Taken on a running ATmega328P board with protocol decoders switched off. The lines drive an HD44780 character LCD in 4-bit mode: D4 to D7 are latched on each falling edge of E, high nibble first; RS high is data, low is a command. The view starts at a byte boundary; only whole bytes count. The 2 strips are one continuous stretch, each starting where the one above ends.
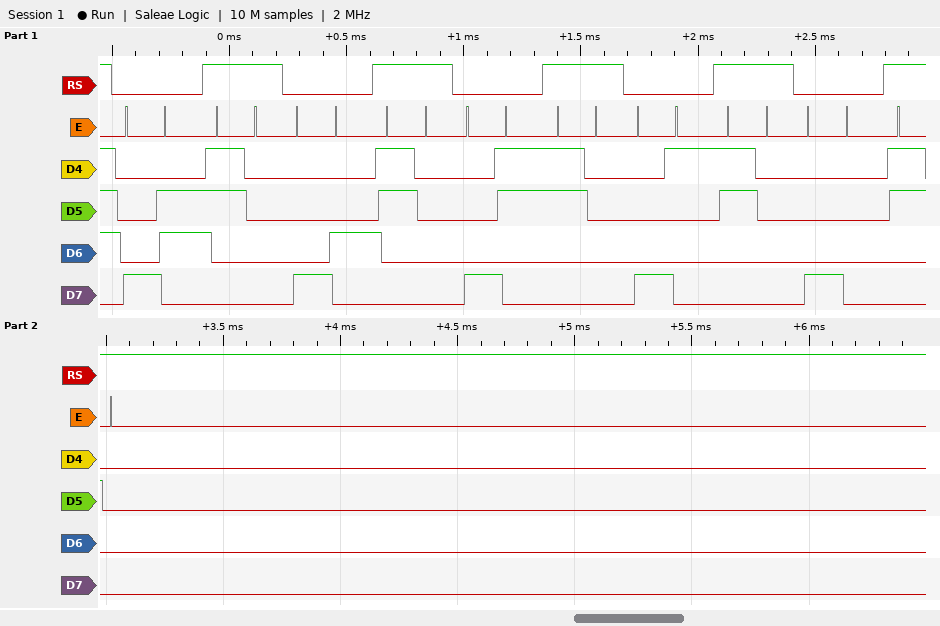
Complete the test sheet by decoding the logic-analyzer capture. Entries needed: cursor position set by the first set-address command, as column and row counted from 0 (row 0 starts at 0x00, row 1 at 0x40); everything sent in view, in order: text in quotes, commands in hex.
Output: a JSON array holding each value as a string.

["column 6, row 0", "0x86 \"0\" 0x84 \"0\" 0x83 \"0\" 0x81 \"0\" 0x80 \"0\""]
